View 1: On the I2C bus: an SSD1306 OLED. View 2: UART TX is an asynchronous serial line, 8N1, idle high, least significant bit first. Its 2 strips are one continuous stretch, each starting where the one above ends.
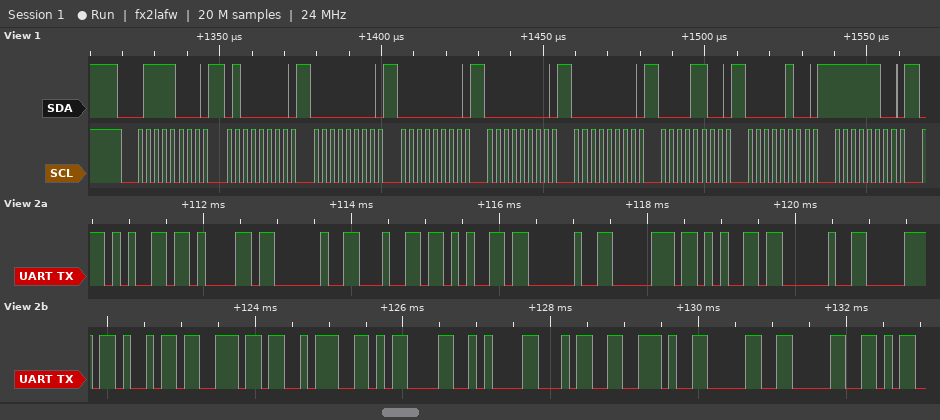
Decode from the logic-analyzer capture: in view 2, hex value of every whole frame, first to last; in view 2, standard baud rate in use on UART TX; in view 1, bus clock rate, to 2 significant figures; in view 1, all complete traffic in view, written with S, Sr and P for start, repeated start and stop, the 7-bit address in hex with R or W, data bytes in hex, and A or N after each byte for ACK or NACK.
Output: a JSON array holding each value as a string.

["65 61 20 64 65 20 70 65 20 70 69 6E 3A 0D 0A 34 2E 30 30", "9600 baud", "400 kHz", "S 3CW A 40 A 00 A 00 A 00 A 00 A 0C A 04 A FC A"]
